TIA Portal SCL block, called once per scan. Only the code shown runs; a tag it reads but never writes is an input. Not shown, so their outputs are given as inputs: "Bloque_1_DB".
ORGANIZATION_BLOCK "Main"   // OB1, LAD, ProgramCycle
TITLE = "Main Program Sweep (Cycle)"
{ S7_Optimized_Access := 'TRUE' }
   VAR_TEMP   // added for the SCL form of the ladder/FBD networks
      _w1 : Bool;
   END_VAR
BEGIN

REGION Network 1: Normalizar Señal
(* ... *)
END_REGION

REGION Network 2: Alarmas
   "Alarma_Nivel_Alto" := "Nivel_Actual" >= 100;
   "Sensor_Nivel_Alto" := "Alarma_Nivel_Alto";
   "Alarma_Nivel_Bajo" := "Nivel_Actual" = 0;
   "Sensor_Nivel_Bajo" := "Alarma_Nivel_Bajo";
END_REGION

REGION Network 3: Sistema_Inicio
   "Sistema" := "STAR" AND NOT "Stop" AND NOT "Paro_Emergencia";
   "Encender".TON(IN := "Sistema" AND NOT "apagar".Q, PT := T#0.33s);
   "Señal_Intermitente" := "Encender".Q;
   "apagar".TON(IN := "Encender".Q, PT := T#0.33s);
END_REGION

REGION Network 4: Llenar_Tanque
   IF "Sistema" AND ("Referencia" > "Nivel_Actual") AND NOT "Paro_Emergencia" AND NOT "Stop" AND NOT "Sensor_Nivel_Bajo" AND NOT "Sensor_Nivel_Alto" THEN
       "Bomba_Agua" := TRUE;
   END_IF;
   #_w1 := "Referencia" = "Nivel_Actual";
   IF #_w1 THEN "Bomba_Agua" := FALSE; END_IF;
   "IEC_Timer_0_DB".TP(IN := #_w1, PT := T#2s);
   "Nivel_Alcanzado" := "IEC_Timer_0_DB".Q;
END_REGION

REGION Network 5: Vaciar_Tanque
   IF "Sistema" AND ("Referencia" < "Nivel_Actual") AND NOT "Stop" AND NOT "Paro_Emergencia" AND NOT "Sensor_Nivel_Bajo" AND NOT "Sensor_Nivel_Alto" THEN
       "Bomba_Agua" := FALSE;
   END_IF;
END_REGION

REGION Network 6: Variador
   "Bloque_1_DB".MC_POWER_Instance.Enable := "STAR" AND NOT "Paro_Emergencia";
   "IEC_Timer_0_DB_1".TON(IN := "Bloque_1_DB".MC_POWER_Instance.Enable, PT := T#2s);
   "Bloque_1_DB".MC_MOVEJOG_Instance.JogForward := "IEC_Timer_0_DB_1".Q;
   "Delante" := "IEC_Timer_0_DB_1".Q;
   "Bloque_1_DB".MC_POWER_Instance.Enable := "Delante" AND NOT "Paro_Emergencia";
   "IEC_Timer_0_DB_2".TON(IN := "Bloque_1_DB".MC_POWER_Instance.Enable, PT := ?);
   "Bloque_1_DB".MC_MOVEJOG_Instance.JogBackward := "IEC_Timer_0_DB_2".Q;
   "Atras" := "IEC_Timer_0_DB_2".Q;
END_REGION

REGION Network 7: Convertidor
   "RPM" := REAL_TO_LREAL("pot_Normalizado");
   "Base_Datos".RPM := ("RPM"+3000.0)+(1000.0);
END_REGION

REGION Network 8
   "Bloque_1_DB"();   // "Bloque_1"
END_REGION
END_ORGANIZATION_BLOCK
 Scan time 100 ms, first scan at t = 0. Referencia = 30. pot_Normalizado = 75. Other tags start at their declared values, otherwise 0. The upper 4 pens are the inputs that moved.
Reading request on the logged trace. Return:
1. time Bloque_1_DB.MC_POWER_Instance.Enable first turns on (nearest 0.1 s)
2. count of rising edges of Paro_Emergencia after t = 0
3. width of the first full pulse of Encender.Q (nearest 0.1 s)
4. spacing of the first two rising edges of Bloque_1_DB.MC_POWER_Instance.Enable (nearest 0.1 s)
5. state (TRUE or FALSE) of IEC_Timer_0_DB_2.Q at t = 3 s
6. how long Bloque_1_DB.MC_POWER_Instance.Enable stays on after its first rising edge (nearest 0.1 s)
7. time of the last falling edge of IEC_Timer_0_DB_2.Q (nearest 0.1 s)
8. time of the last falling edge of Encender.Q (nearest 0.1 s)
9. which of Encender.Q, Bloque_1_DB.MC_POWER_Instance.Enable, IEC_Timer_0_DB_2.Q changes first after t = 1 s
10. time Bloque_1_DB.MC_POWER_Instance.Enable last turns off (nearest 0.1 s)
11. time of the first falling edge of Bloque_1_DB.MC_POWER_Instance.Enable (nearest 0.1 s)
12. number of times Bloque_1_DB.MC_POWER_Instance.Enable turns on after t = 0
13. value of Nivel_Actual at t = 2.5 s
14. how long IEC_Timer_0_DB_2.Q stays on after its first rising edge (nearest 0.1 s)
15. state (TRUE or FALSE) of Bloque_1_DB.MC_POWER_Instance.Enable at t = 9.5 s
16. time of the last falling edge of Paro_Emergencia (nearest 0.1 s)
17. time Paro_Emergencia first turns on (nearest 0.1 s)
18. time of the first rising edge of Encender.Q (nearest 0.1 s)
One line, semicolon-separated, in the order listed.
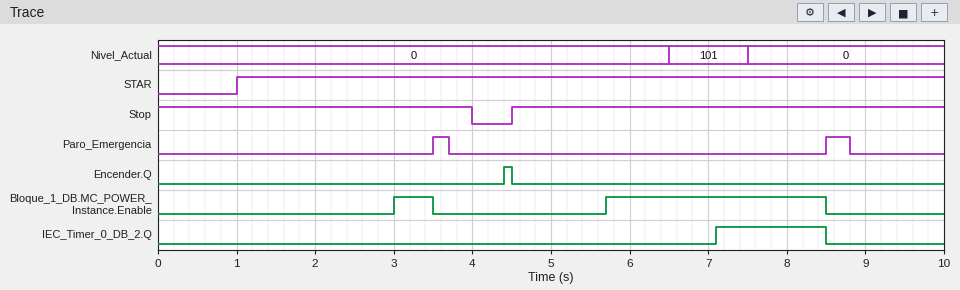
3.0 s; 2; 0.1 s; 2.7 s; FALSE; 0.5 s; 8.5 s; 4.5 s; Bloque_1_DB.MC_POWER_Instance.Enable; 8.5 s; 3.5 s; 2; 0; 1.4 s; FALSE; 8.8 s; 3.5 s; 4.4 s
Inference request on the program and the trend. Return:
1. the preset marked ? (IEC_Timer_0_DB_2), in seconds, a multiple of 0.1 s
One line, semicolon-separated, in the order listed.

1.4 s
